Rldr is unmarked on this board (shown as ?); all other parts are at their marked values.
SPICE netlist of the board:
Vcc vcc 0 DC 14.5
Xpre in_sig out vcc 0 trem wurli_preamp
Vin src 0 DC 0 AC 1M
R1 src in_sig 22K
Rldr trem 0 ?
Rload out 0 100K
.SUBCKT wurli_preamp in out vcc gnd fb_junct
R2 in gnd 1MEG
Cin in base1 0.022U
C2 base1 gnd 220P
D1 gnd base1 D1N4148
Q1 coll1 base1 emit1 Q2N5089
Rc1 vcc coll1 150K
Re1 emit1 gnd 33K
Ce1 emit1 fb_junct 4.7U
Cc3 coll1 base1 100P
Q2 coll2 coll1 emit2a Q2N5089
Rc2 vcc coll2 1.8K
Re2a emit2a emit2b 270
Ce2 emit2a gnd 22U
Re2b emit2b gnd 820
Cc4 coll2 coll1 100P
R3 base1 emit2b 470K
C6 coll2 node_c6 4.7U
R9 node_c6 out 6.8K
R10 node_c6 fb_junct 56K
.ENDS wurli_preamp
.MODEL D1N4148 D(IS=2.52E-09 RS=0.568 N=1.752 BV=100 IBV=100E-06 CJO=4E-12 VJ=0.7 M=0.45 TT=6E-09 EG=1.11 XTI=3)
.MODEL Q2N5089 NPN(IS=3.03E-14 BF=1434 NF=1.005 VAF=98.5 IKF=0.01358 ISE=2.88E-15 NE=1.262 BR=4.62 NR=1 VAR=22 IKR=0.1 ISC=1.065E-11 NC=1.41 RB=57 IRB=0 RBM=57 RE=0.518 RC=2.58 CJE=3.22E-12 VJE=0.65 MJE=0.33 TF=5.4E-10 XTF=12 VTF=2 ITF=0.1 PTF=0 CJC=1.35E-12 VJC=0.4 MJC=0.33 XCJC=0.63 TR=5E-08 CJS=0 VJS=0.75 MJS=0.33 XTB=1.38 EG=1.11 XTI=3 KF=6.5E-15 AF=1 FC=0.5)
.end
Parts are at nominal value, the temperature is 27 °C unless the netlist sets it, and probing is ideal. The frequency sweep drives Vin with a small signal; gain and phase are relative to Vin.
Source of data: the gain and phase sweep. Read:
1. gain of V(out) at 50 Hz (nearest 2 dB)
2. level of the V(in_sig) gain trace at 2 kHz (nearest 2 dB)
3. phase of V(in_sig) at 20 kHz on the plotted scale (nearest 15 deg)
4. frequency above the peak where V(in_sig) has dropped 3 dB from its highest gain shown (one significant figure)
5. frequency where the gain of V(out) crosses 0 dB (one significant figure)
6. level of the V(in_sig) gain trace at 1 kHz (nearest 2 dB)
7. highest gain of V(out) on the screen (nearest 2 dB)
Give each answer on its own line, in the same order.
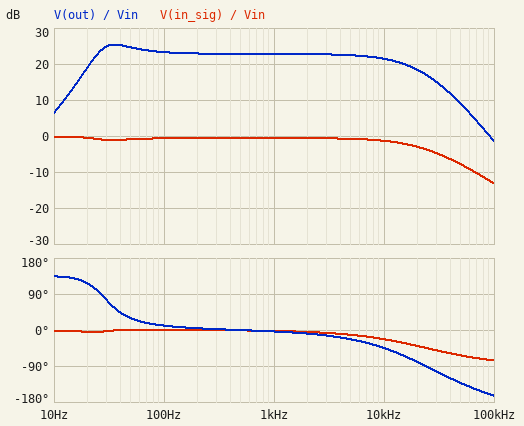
24 dB
0 dB
-45 deg
20 kHz
90 kHz
0 dB
26 dB
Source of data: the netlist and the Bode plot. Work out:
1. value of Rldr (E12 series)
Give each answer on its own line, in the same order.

3.9 kΩ
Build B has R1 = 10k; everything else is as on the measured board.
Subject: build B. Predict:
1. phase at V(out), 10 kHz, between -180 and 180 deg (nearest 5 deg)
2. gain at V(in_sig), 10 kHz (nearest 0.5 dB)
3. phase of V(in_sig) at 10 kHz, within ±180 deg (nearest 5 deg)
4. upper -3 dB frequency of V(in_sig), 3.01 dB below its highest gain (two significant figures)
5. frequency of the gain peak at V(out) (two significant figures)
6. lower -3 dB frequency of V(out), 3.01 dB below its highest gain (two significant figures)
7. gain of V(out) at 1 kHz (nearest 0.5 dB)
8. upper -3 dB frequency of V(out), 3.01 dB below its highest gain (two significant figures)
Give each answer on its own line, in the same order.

-35 deg
-0.5 dB
-10 deg
48 kHz
35 Hz
25 Hz
23.0 dB
3.5 kHz
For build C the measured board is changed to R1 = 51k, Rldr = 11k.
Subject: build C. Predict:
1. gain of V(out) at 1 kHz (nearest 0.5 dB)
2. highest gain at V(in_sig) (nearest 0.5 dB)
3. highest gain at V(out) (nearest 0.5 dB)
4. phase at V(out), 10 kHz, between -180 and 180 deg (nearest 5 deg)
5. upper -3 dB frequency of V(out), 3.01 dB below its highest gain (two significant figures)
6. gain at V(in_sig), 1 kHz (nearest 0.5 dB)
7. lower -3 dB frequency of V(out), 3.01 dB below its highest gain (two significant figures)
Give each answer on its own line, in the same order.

15.5 dB
-0.5 dB
16.0 dB
-65 deg
8.2 kHz
-1.5 dB
17 Hz
